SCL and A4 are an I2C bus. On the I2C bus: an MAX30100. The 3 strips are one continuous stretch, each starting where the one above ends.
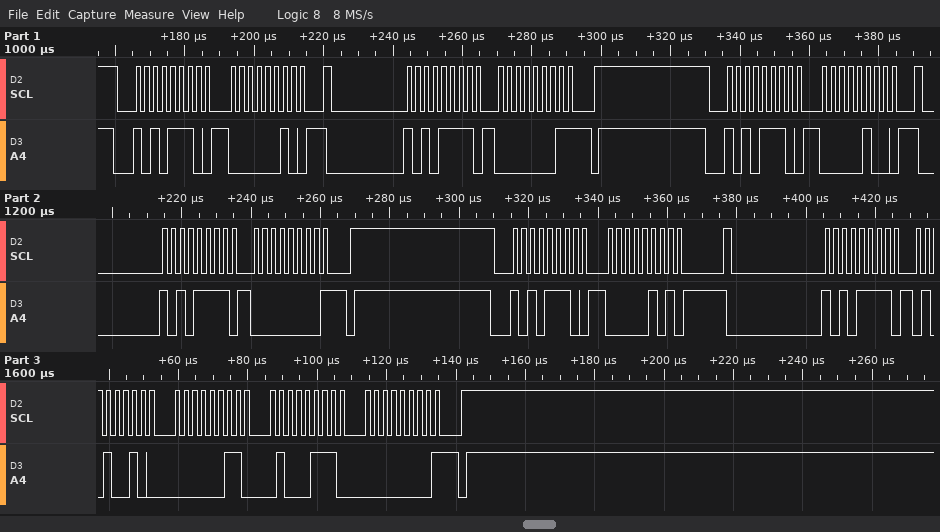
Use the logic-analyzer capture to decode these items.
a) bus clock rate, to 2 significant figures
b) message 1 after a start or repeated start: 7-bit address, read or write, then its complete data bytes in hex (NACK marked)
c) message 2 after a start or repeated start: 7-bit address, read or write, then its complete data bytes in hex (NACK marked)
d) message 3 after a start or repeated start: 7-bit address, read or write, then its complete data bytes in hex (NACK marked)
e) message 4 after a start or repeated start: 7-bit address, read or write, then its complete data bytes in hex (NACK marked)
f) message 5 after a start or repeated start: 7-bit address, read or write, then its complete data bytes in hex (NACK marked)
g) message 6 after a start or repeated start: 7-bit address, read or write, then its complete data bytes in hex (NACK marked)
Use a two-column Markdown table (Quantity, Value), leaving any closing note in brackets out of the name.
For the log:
| Quantity | Value |
|---|---|
| bus clock rate, to 2 significant figures | 400 kHz |
| message 1 after a start or repeated start: 7-bit address, read or write, then its complete data bytes in hex | 0x57 write: 02 |
| message 2 after a start or repeated start: 7-bit address, read or write, then its complete data bytes in hex | 0x57 read: 01 NACK |
| message 3 after a start or repeated start: 7-bit address, read or write, then its complete data bytes in hex | 0x57 write: 04 |
| message 4 after a start or repeated start: 7-bit address, read or write, then its complete data bytes in hex | 0x57 read: 00 NACK |
| message 5 after a start or repeated start: 7-bit address, read or write, then its complete data bytes in hex | 0x57 write: 05 |
| message 6 after a start or repeated start: 7-bit address, read or write, then its complete data bytes in hex | 0x57 read: 52 03 47 00 NACK |
